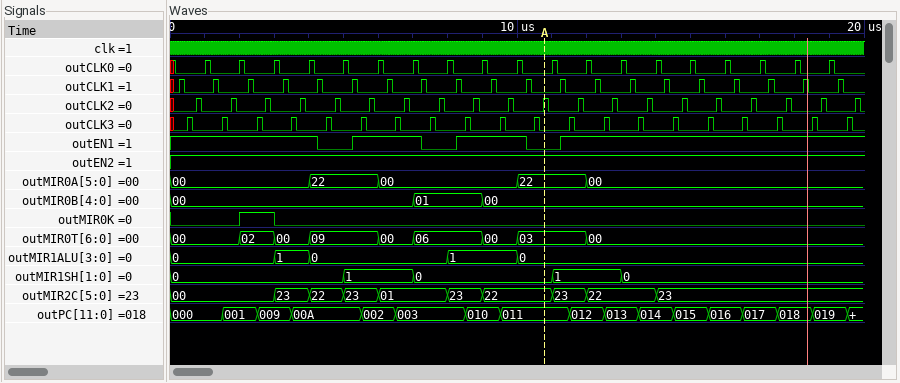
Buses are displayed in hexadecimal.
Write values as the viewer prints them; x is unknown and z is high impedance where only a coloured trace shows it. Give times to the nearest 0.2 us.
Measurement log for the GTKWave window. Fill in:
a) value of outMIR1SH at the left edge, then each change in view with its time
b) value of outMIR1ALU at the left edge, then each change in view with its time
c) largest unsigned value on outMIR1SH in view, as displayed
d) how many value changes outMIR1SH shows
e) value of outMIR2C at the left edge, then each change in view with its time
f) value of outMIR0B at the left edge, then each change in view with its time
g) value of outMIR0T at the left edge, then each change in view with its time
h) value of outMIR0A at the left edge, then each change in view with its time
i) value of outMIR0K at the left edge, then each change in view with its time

0, 1 at 5 us, 0 at 7 us, 1 at 11 us, 0 at 13 us
0, 1 at 3 us, 0 at 4 us, 1 at 8 us, 0 at 10 us
1
4
00, 23 at 3 us, 22 at 4 us, 23 at 5 us, 01 at 6 us, 23 at 8 us, 22 at 9 us, 23 at 11 us, 22 at 12 us, 23 at 14 us
00, 01 at 7 us, 00 at 9 us
00, 02 at 2 us, 00 at 3 us, 09 at 4 us, 00 at 6 us, 06 at 7 us, 00 at 9 us, 03 at 10 us, 00 at 12 us
00, 22 at 4 us, 00 at 6 us, 22 at 10 us, 00 at 12 us
0, 1 at 2 us, 0 at 3 us
